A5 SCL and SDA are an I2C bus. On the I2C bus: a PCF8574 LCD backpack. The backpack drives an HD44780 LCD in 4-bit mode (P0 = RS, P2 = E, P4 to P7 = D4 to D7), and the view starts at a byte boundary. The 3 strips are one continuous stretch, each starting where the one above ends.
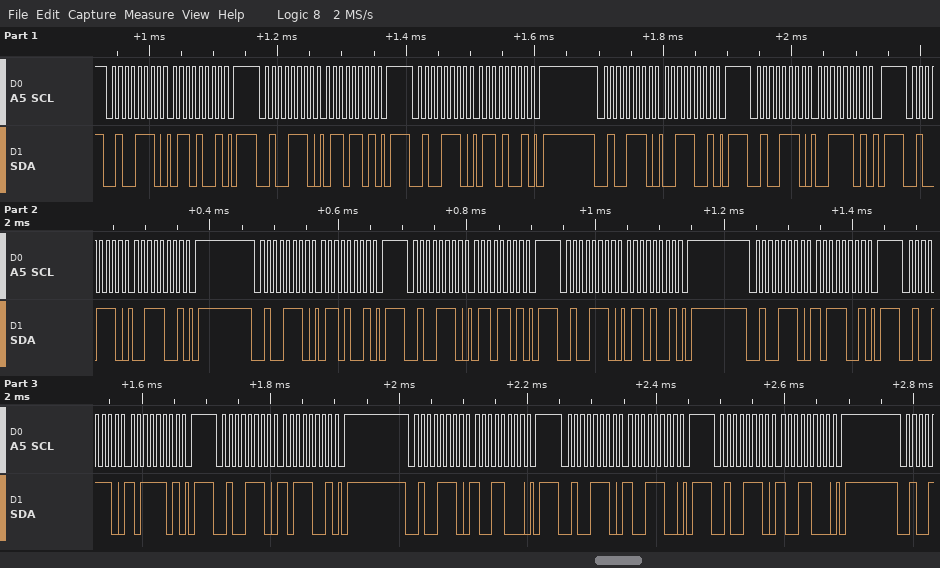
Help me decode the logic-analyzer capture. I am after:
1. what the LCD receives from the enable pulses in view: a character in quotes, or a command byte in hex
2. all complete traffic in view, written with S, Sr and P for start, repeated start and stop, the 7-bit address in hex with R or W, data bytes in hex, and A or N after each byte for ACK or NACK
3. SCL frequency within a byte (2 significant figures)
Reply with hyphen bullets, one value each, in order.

- 'c' 'k'
- S 27W A 69 A P S 27W A 6D A P S 27W A 69 A P S 27W A 39 A P S 27W A 3D A P S 27W A 39 A P S 27W A 69 A P S 27W A 6D A P S 27W A 69 A P S 27W A B9 A P S 27W A BD A P S 27W A B9 A P S 27W A 98 A P S 27W A 9C A P S 27W A 98 A P
- 100 kHz
